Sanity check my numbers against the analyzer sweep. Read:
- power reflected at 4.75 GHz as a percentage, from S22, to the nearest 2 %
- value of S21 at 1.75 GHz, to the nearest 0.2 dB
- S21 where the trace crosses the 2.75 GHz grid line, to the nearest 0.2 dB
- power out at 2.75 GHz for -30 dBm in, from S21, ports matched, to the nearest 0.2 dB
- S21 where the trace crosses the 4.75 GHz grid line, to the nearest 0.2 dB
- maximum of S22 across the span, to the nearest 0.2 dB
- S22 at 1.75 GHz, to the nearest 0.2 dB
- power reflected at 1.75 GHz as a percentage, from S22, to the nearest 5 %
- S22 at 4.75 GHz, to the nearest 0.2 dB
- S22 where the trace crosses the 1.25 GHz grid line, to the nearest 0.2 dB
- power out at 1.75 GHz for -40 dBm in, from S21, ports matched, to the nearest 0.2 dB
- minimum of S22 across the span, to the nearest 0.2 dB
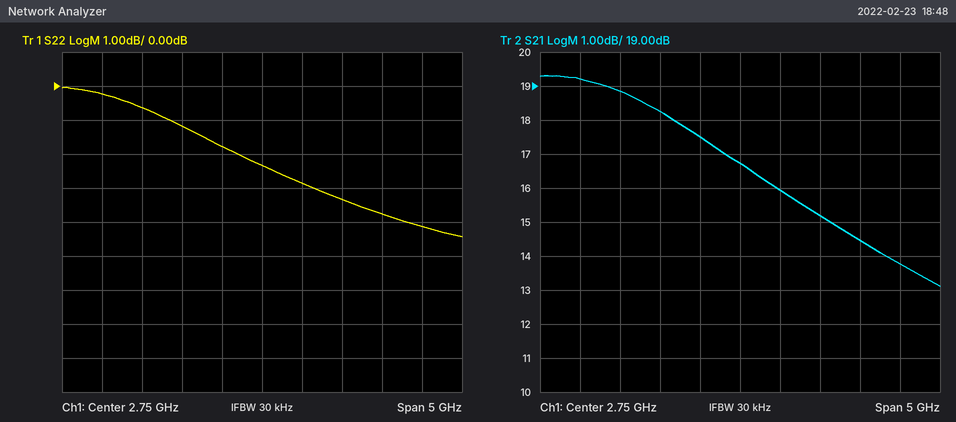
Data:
38 %
18.2 dB
16.8 dB
-13.2 dBm
13.8 dB
0.0 dB
-1.2 dB
75 %
-4.2 dB
-0.6 dB
-21.8 dBm
-4.4 dB
